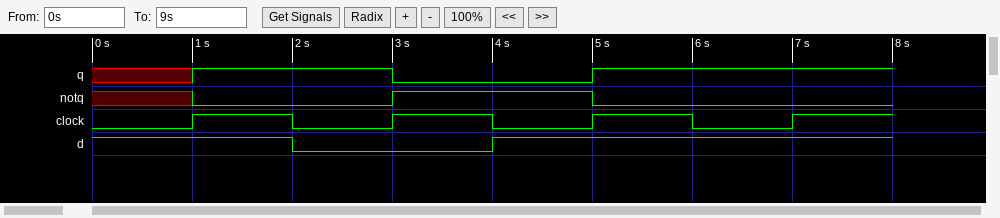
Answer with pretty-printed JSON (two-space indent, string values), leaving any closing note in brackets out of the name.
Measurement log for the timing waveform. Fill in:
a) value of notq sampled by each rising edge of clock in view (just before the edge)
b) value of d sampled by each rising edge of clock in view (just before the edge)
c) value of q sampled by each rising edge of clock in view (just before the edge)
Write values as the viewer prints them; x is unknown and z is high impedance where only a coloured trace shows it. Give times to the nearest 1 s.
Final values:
{
  "value of notq sampled by each rising edge of clock in view": "x 0 1 0",
  "value of d sampled by each rising edge of clock in view": "1 0 1 1",
  "value of q sampled by each rising edge of clock in view": "x 1 0 1"
}
